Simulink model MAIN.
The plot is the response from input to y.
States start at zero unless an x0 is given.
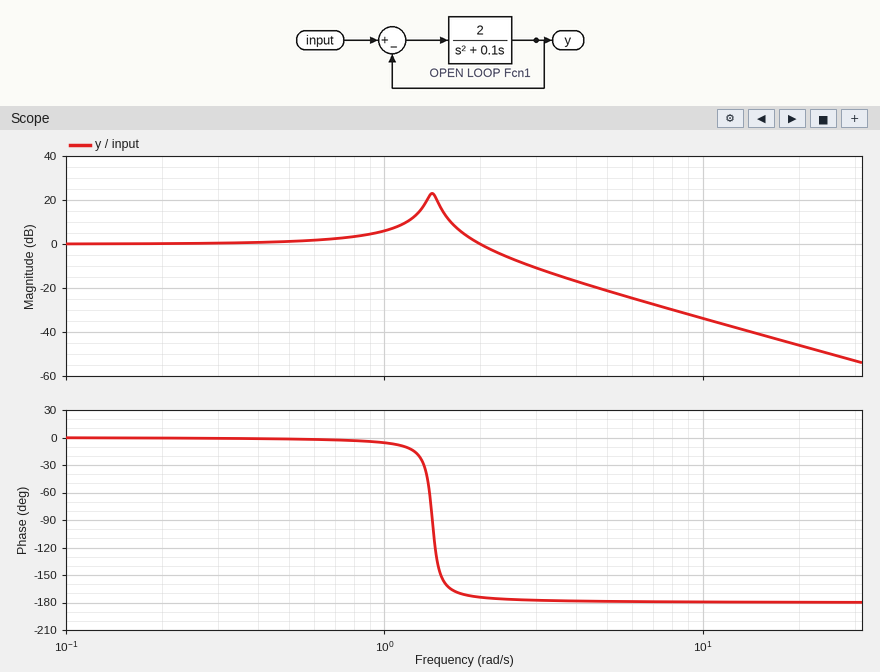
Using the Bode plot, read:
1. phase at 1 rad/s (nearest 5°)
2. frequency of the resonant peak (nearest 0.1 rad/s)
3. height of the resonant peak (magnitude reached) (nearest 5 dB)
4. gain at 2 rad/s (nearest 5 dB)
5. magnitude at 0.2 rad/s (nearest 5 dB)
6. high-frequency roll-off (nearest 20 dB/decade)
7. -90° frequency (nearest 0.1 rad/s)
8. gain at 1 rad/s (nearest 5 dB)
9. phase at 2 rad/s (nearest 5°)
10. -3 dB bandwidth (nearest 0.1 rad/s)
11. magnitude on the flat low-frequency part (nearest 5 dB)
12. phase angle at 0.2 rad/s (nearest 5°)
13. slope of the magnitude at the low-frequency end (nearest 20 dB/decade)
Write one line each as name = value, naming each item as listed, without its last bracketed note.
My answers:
phase at 1 rad/s = -5°
frequency of the resonant peak = 1.4 rad/s
height of the resonant peak (magnitude reached) = 25 dB
gain at 2 rad/s = 0 dB
magnitude at 0.2 rad/s = 0 dB
high-frequency roll-off = -40 dB/decade
-90° frequency = 1.4 rad/s
gain at 1 rad/s = 5 dB
phase at 2 rad/s = -175°
-3 dB bandwidth = 2.2 rad/s
magnitude on the flat low-frequency part = 0 dB
phase angle at 0.2 rad/s = 0°
slope of the magnitude at the low-frequency end = 0 dB/decade
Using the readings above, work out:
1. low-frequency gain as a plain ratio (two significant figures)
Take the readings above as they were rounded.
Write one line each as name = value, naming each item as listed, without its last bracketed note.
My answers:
low-frequency gain as a plain ratio = 1.0
